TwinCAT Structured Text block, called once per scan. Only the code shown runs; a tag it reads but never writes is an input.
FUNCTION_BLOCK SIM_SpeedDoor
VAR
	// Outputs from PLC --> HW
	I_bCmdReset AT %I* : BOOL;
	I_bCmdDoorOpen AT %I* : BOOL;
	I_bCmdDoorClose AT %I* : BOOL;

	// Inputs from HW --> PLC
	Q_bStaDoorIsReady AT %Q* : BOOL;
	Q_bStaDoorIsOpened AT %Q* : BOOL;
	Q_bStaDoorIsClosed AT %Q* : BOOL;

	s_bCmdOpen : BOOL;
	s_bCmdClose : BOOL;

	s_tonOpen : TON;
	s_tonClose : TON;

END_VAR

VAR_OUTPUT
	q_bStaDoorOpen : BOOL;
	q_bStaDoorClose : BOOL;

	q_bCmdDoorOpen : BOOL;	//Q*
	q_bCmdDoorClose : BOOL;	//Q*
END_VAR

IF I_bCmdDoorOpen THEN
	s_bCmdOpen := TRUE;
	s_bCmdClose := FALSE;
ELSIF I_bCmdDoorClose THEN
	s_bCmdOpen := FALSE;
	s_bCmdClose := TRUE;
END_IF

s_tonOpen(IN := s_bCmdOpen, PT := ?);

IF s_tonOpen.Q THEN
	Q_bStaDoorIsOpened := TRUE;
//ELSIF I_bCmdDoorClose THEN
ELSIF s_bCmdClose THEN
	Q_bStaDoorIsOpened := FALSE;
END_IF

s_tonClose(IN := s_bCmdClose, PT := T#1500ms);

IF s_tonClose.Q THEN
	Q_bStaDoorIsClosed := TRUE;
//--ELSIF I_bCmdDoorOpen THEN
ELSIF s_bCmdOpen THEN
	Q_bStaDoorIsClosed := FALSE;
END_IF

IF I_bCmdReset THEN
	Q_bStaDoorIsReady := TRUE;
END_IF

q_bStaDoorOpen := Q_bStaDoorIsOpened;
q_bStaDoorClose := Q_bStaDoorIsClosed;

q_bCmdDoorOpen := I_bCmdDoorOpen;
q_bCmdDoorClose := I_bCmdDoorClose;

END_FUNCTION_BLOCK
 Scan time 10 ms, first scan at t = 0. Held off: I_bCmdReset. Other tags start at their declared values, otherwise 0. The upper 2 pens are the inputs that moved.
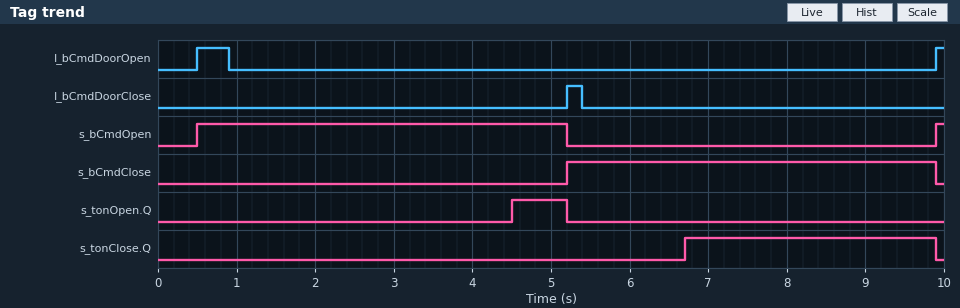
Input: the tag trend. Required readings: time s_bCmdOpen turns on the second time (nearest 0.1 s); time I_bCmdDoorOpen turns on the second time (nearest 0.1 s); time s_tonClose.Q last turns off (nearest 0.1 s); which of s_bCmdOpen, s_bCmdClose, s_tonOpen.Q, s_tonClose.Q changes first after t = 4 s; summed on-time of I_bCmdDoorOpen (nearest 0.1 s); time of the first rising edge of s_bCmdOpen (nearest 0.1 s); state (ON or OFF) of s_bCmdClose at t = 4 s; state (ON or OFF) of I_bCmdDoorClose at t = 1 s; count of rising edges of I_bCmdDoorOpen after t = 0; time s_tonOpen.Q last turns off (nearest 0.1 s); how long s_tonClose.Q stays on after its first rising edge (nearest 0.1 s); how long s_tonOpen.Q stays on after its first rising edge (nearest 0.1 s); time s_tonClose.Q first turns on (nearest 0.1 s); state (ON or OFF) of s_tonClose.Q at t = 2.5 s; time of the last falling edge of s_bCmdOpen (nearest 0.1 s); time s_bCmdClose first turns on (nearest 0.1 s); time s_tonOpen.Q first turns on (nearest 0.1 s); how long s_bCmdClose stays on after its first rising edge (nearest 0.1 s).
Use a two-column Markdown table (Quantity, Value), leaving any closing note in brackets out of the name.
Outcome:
| Quantity | Value |
|---|---|
| time s_bCmdOpen turns on the second time | 9.9 s |
| time I_bCmdDoorOpen turns on the second time | 9.9 s |
| time s_tonClose.Q last turns off | 9.9 s |
| which of s_bCmdOpen, s_bCmdClose, s_tonOpen.Q, s_tonClose.Q changes first after t = 4 s | s_tonOpen.Q |
| summed on-time of I_bCmdDoorOpen | 0.5 s |
| time of the first rising edge of s_bCmdOpen | 0.5 s |
| state (ON or OFF) of s_bCmdClose at t = 4 s | OFF |
| state (ON or OFF) of I_bCmdDoorClose at t = 1 s | OFF |
| count of rising edges of I_bCmdDoorOpen after t = 0 | 2 |
| time s_tonOpen.Q last turns off | 5.2 s |
| how long s_tonClose.Q stays on after its first rising edge | 3.2 s |
| how long s_tonOpen.Q stays on after its first rising edge | 0.7 s |
| time s_tonClose.Q first turns on | 6.7 s |
| state (ON or OFF) of s_tonClose.Q at t = 2.5 s | OFF |
| time of the last falling edge of s_bCmdOpen | 5.2 s |
| time s_bCmdClose first turns on | 5.2 s |
| time s_tonOpen.Q first turns on | 4.5 s |
| how long s_bCmdClose stays on after its first rising edge | 4.7 s |
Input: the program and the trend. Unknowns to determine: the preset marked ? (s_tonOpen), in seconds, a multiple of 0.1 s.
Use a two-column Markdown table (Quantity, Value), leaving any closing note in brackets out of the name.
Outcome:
| Quantity | Value |
|---|---|
| the preset marked ? (s_tonOpen), in seconds, a multiple of 0.1 s | 4.0 s |
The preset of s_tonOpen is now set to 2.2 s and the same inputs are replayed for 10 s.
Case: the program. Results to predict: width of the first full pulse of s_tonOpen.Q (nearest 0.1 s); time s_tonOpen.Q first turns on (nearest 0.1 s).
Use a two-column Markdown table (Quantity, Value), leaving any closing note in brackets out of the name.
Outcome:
| Quantity | Value |
|---|---|
| width of the first full pulse of s_tonOpen.Q | 2.5 s |
| time s_tonOpen.Q first turns on | 2.7 s |
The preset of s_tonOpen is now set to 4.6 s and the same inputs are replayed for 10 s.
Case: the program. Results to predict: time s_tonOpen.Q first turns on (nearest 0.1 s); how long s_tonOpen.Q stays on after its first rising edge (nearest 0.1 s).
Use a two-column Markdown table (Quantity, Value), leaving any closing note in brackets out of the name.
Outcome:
| Quantity | Value |
|---|---|
| time s_tonOpen.Q first turns on | 5.1 s |
| how long s_tonOpen.Q stays on after its first rising edge | 0.1 s |
